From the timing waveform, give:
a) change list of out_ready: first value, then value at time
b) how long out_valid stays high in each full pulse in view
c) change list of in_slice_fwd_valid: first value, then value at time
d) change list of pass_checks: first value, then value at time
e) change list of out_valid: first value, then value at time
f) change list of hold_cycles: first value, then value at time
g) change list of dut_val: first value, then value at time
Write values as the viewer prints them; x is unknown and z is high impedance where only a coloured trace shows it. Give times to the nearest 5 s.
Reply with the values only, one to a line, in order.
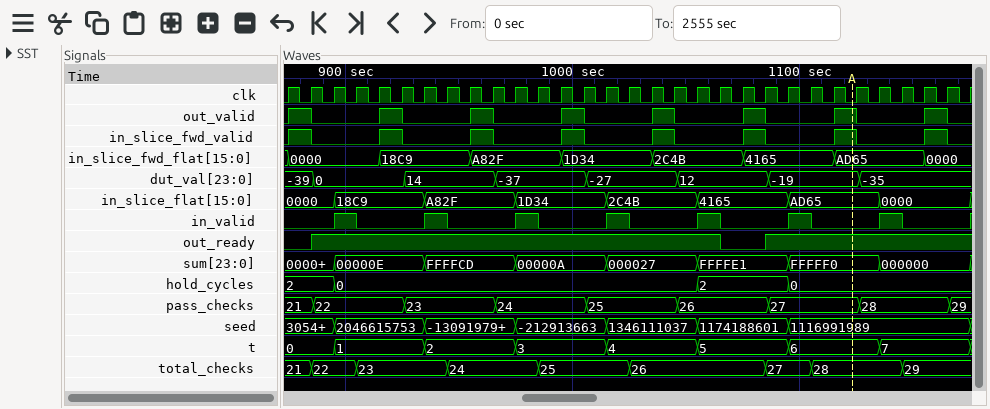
0, 1 at 885 s, 0 at 1065 s, 1 at 1085 s
10 s, 10 s, 10 s, 10 s, 10 s, 10 s, 10 s, 10 s
0, 1 at 875 s, 0 at 885 s, 1 at 915 s, 0 at 925 s, 1 at 955 s, 0 at 965 s, 1 at 995 s, 0 at 1005 s, 1 at 1035 s, 0 at 1045 s, 1 at 1075 s, 0 at 1085 s, 1 at 1115 s, 0 at 1125 s, 1 at 1155 s, 0 at 1165 s
21, 22 at 885 s, 23 at 925 s, 24 at 965 s, 25 at 1005 s, 26 at 1045 s, 27 at 1085 s, 28 at 1125 s, 29 at 1165 s
0, 1 at 875 s, 0 at 885 s, 1 at 915 s, 0 at 925 s, 1 at 955 s, 0 at 965 s, 1 at 995 s, 0 at 1005 s, 1 at 1035 s, 0 at 1045 s, 1 at 1075 s, 0 at 1085 s, 1 at 1115 s, 0 at 1125 s, 1 at 1155 s, 0 at 1165 s
2, 0 at 895 s, 2 at 1055 s, 0 at 1095 s
-39, 0 at 885 s, 14 at 925 s, -37 at 965 s, -27 at 1005 s, 12 at 1045 s, -19 at 1085 s, -35 at 1125 s
